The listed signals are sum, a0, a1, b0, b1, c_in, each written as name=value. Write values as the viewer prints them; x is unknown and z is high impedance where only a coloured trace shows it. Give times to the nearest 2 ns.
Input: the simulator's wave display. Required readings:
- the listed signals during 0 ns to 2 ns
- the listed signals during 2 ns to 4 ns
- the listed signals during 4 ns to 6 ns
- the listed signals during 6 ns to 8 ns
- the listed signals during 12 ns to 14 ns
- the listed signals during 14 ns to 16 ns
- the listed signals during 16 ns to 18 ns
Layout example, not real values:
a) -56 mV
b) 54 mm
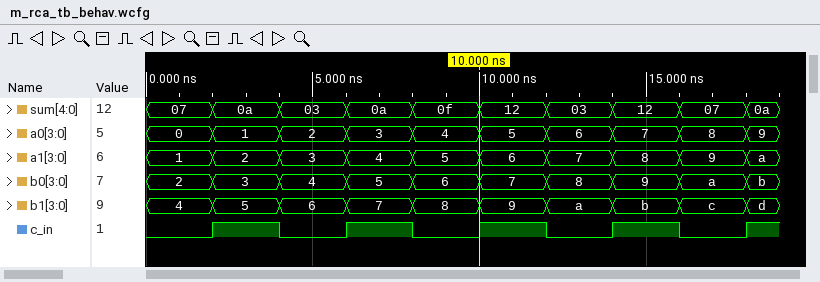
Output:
a) sum=07, a0=0, a1=1, b0=2, b1=4, c_in=0
b) sum=0a, a0=1, a1=2, b0=3, b1=5, c_in=1
c) sum=03, a0=2, a1=3, b0=4, b1=6, c_in=0
d) sum=0a, a0=3, a1=4, b0=5, b1=7, c_in=1
e) sum=03, a0=6, a1=7, b0=8, b1=a, c_in=0
f) sum=12, a0=7, a1=8, b0=9, b1=b, c_in=1
g) sum=07, a0=8, a1=9, b0=a, b1=c, c_in=0
